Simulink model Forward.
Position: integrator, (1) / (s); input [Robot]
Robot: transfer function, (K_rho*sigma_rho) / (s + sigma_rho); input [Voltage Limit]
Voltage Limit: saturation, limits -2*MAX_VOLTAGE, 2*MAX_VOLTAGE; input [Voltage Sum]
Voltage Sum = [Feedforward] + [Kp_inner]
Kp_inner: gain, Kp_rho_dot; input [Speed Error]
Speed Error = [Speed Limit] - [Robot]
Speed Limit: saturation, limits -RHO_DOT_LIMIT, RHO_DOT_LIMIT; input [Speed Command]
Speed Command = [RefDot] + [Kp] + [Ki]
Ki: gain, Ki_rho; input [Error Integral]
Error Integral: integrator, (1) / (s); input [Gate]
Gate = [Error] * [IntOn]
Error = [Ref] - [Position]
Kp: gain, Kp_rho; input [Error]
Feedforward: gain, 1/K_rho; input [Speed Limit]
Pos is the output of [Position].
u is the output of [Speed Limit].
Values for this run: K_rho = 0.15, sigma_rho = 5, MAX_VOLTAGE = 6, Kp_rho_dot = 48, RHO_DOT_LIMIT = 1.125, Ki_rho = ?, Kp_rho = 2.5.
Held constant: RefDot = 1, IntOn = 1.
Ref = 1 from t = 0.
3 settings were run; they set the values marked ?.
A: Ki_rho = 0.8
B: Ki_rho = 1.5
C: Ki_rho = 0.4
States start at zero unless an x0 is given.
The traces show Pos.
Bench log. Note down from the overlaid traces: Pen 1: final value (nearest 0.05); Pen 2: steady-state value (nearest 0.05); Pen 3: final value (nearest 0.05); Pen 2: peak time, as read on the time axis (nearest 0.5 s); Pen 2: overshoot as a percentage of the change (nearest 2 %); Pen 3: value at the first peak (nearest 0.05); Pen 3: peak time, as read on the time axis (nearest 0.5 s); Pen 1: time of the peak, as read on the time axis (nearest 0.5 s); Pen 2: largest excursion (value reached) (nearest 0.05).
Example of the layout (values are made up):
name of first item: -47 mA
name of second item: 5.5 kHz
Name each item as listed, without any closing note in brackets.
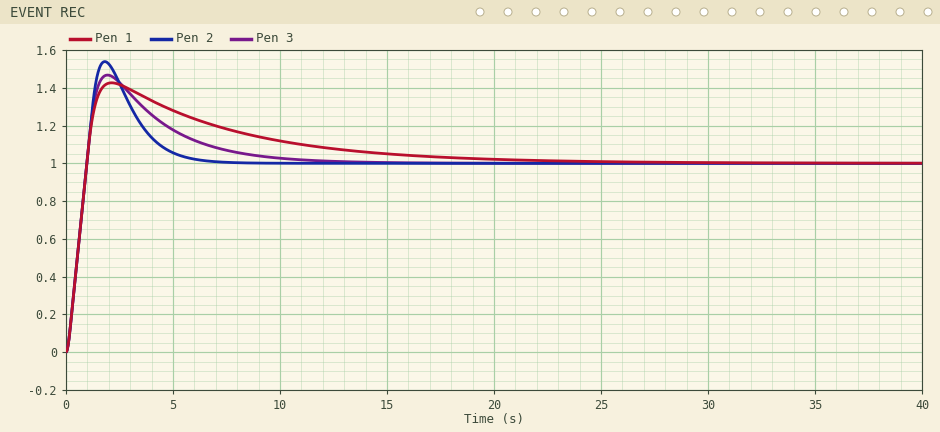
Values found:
Pen 1: final value: 1.00
Pen 2: steady-state value: 1.00
Pen 3: final value: 1.00
Pen 2: peak time, as read on the time axis: 2.0 s
Pen 2: overshoot as a percentage of the change: 54 %
Pen 3: value at the first peak: 1.45
Pen 3: peak time, as read on the time axis: 2.0 s
Pen 1: time of the peak, as read on the time axis: 2.0 s
Pen 2: largest excursion (value reached): 1.55
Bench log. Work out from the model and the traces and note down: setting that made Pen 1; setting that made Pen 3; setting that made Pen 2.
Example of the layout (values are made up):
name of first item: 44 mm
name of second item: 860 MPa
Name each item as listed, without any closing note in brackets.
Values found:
setting that made Pen 1: C
setting that made Pen 3: A
setting that made Pen 2: B
